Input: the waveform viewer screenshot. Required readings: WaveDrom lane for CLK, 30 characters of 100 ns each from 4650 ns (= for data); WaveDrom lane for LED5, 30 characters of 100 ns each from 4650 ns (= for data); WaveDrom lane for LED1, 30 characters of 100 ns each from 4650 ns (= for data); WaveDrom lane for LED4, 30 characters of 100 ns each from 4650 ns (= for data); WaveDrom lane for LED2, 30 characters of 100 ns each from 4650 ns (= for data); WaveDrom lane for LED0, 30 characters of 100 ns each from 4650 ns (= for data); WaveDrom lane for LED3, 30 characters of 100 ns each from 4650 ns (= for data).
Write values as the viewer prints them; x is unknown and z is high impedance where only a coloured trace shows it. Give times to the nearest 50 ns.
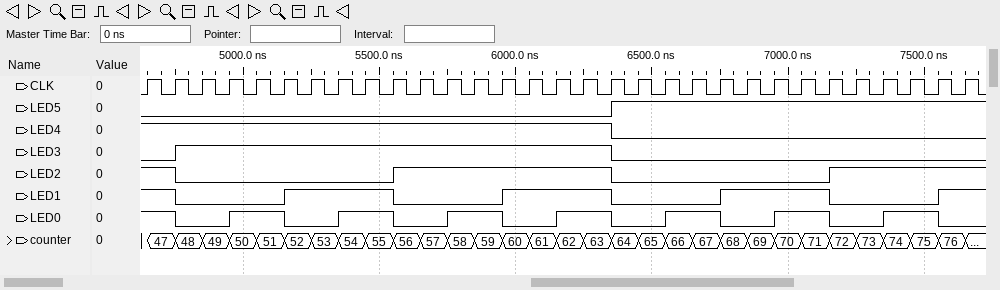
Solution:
{name: 'CLK', wave: 'p.............................'}
{name: 'LED5', wave: '0................1............'}
{name: 'LED1', wave: '10...1...0...1...0...1...0...1'}
{name: 'LED4', wave: '1................0............'}
{name: 'LED2', wave: '10.......1.......0.......1....'}
{name: 'LED0', wave: '10.1.0.1.0.1.0.1.0.1.0.1.0.1.0'}
{name: 'LED3', wave: '01...............0............'}
